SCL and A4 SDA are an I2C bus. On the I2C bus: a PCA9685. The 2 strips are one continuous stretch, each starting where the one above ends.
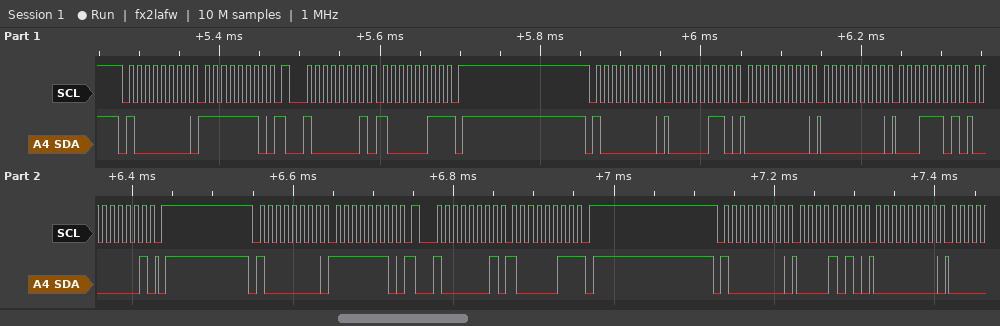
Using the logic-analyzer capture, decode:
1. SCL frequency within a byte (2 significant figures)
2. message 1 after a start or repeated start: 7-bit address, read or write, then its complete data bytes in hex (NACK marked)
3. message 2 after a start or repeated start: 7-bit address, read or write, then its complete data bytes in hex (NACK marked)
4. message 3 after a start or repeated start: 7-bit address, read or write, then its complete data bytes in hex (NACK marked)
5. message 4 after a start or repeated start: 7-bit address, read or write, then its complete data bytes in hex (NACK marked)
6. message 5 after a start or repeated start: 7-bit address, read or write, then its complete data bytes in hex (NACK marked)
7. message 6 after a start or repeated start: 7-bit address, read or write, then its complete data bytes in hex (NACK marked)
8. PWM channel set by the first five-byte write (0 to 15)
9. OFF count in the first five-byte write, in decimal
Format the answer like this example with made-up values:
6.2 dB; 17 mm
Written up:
100 kHz; 0x40 write: FE; 0x40 read: 83 NACK; 0x40 write: 06 00 00 1D 01; 0x40 write: FE; 0x40 read: 83 NACK; 0x40 write: 0A 00; 0; 285
